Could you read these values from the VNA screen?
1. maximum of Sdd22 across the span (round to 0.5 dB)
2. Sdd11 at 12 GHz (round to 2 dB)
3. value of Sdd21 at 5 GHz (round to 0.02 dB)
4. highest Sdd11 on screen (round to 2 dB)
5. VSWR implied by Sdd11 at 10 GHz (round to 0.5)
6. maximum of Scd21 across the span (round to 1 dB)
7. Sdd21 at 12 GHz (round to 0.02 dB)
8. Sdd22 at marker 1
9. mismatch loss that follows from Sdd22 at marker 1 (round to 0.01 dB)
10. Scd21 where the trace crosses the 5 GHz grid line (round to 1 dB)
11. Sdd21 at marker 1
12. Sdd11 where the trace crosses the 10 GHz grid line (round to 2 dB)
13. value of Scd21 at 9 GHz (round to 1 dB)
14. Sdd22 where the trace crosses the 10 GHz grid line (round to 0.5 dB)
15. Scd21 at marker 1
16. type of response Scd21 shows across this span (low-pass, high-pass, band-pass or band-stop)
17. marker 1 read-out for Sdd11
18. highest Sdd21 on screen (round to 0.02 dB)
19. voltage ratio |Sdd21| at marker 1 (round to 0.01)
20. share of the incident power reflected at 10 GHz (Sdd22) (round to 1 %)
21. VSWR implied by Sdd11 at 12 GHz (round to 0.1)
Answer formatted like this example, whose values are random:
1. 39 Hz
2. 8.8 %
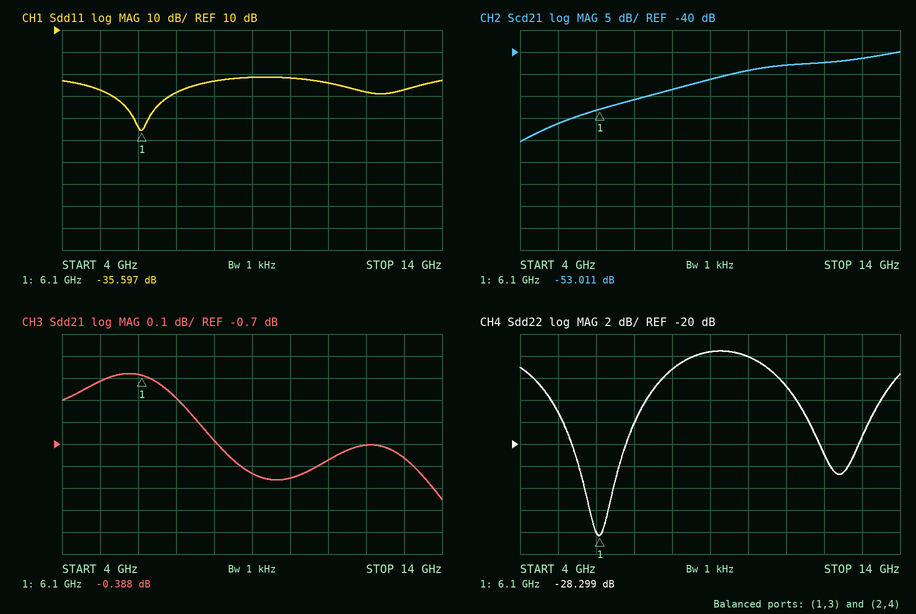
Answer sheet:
1. -11.5 dB
2. -18 dB
3. -0.42 dB
4. -12 dB
5. 1.5
6. -40 dB
7. -0.70 dB
8. -28.299 dB
9. 0.01 dB
10. -56 dB
11. -0.388 dB
12. -12 dB
13. -46 dB
14. -12.0 dB
15. -53.011 dB
16. high-pass
17. -35.597 dB
18. -0.38 dB
19. 0.96
20. 6 %
21. 1.3
